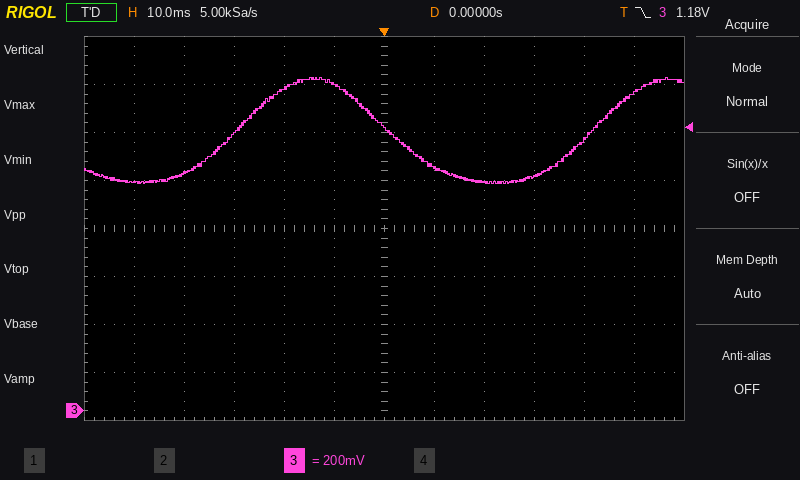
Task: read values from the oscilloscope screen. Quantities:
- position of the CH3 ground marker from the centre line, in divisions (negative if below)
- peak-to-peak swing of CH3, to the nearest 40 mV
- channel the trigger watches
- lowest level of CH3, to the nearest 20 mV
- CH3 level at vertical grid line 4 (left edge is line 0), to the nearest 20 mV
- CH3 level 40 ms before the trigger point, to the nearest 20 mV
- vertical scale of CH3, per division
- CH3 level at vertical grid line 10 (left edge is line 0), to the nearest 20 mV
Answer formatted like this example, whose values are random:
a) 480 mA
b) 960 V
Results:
a) -3.8 div
b) 440 mV
c) CH3
d) 940 mV
e) 1.34 V
f) 980 mV
g) 200 mV
h) 1.12 V
